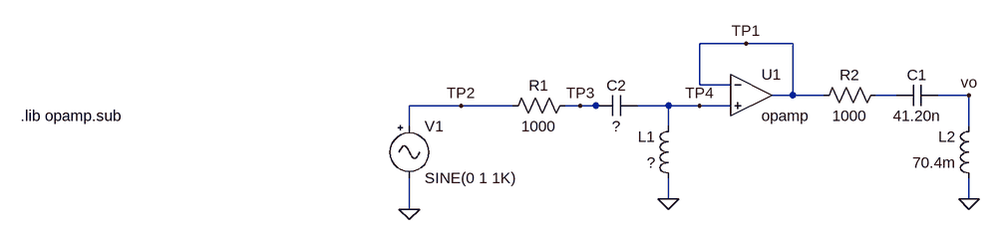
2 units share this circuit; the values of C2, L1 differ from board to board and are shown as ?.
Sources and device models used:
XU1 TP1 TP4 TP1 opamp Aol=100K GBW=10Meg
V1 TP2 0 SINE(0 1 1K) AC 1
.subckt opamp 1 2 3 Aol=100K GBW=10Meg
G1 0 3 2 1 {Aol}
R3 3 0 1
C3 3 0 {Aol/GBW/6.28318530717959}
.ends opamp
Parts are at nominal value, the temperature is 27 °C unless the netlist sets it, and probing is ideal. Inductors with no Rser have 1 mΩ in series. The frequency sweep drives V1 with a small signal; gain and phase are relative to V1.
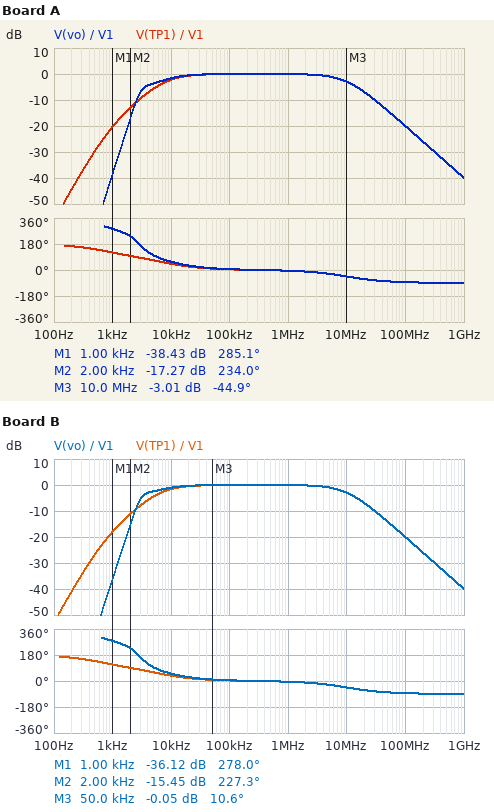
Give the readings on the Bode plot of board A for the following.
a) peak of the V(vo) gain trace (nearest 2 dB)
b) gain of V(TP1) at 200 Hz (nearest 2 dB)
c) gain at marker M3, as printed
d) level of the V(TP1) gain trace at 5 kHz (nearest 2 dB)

0 dB
-44 dB
-3.01 dB
-6 dB
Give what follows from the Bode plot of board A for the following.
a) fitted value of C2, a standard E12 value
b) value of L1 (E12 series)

220 nF
18 mH
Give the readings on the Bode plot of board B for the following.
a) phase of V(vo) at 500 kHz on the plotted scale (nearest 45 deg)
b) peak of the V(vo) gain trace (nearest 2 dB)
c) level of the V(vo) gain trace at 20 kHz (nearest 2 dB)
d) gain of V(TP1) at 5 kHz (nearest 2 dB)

0 deg
0 dB
0 dB
-4 dB
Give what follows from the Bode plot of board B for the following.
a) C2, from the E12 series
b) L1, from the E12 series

270 nF
22 mH
